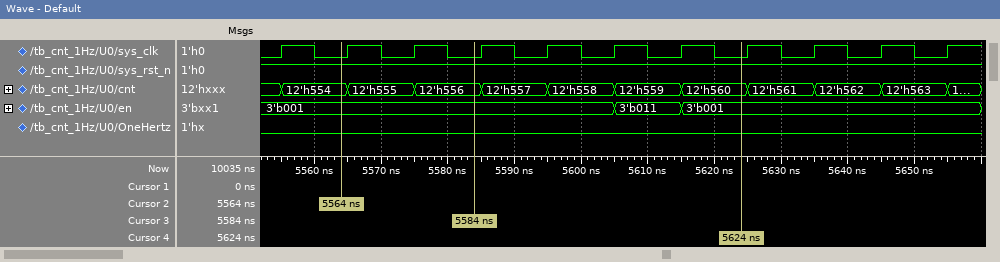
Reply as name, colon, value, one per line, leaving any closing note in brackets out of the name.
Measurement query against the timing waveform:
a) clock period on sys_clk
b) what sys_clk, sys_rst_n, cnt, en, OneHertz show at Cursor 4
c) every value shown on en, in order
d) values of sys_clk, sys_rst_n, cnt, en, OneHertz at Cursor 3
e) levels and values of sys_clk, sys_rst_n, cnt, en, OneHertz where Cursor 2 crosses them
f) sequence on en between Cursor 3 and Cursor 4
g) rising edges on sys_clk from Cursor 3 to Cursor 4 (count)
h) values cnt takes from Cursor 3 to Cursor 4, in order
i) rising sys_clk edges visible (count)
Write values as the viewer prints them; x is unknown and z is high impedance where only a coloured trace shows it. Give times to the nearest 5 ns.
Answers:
clock period on sys_clk: 10 ns
what sys_clk, sys_rst_n, cnt, en, OneHertz show at Cursor 4: sys_clk=0, sys_rst_n=1, cnt=12'h560, en=3'b001, OneHertz=0
every value shown on en, in order: 3'b001, 3'b011, 3'b001
values of sys_clk, sys_rst_n, cnt, en, OneHertz at Cursor 3: sys_clk=0, sys_rst_n=1, cnt=12'h556, en=3'b001, OneHertz=0
levels and values of sys_clk, sys_rst_n, cnt, en, OneHertz where Cursor 2 crosses them: sys_clk=0, sys_rst_n=1, cnt=12'h554, en=3'b001, OneHertz=0
sequence on en between Cursor 3 and Cursor 4: 3'b001, 3'b011, 3'b001
rising edges on sys_clk from Cursor 3 to Cursor 4: 4
values cnt takes from Cursor 3 to Cursor 4, in order: 12'h556, 12'h557, 12'h558, 12'h559, 12'h560
rising sys_clk edges visible: 11
